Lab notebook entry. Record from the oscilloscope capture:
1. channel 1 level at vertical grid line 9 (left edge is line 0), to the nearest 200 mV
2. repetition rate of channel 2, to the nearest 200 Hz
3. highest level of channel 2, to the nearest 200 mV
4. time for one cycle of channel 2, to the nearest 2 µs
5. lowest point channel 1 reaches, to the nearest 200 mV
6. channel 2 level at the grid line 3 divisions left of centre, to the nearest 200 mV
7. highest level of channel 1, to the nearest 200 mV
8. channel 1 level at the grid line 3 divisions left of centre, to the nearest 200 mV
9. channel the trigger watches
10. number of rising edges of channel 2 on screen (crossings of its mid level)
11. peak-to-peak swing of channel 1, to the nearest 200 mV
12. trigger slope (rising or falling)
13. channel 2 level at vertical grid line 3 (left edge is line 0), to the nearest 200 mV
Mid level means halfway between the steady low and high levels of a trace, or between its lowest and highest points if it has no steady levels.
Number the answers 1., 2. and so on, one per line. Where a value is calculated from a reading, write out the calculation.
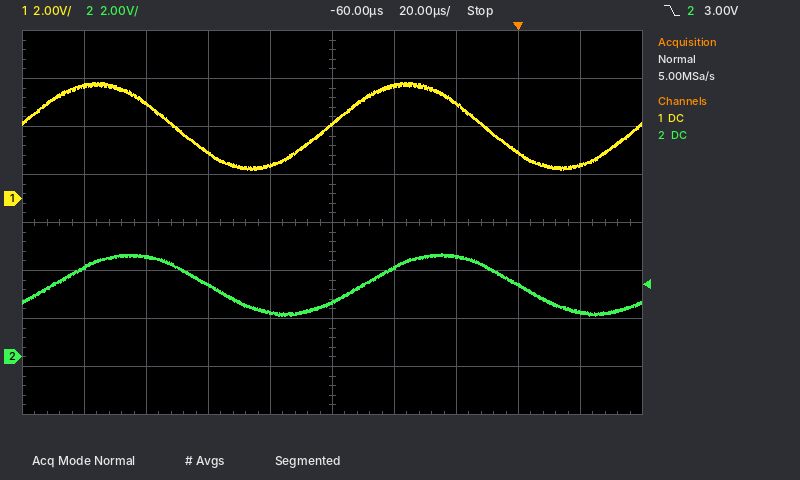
1. 1.4 V
2. 1 / 100 µs ≈ 10.0 kHz
3. 4.4 V
4. 100 µs
5. 1.2 V
6. 4.2 V
7. 4.8 V
8. 4.0 V
9. channel 2
10. 2
11. 4.8 V − (1.2 V) = 3.6 V
12. falling
13. 3.0 V
